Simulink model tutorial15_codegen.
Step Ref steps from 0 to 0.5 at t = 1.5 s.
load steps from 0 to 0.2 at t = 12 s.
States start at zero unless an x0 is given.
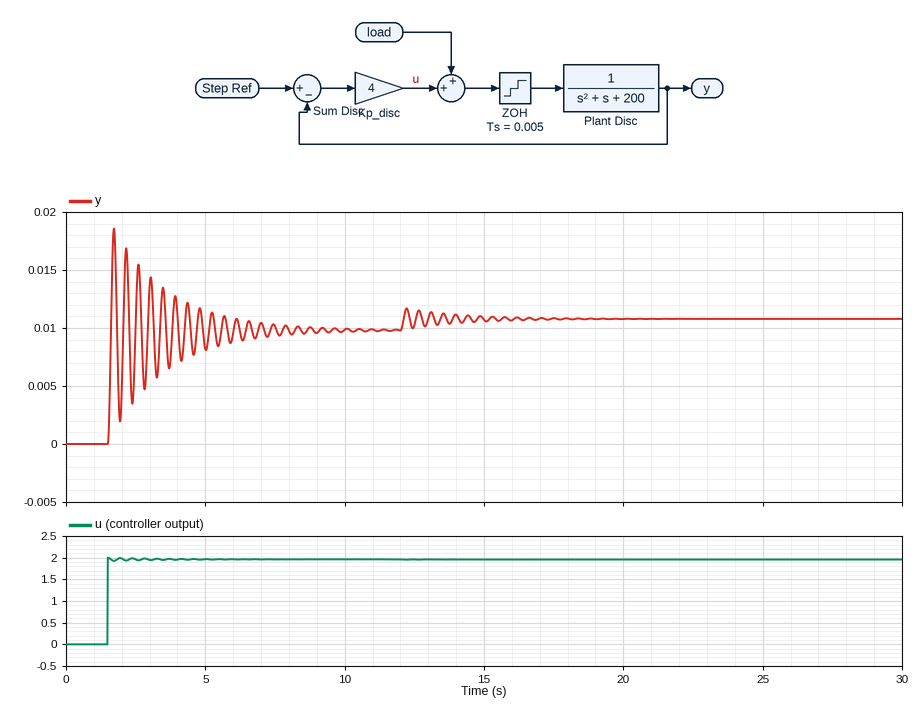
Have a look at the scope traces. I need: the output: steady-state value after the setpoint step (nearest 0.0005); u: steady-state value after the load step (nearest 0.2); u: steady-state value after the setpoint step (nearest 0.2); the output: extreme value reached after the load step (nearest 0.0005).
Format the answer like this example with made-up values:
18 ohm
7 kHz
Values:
0.0100
2.0
2.0
0.0115
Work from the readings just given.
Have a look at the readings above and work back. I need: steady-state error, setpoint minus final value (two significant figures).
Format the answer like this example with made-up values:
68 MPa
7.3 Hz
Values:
0.49
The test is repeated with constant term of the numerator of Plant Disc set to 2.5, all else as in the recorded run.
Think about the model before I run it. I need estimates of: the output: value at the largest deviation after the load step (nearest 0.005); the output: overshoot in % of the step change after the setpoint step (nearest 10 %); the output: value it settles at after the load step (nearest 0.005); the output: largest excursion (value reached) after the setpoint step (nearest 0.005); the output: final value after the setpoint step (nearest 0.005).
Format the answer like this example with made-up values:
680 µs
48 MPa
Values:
0.030
90 %
0.025
0.045
0.025
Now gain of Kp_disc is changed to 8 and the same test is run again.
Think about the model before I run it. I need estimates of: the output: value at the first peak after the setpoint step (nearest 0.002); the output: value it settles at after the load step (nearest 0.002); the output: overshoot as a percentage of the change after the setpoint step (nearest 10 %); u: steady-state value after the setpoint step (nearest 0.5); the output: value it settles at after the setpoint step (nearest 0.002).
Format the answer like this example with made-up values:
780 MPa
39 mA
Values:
0.036
0.020
90 %
4.0
0.020
